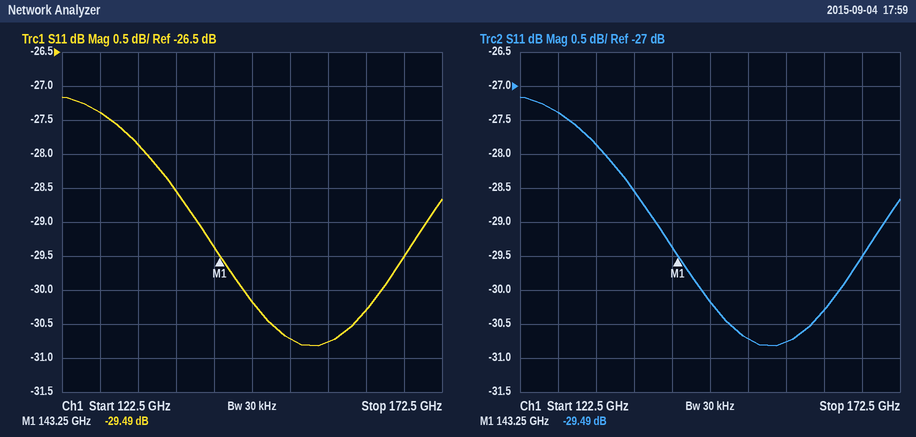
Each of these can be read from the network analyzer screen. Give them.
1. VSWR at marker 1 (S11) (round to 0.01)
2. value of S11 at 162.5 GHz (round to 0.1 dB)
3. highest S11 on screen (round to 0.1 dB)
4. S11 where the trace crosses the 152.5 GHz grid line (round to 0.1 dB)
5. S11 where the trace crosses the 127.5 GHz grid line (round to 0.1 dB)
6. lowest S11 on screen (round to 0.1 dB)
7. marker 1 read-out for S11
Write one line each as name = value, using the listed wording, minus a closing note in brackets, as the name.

VSWR at marker 1 (S11) = 1.07
value of S11 at 162.5 GHz = -30.3 dB
highest S11 on screen = -27.2 dB
S11 where the trace crosses the 152.5 GHz grid line = -30.7 dB
S11 where the trace crosses the 127.5 GHz grid line = -27.4 dB
lowest S11 on screen = -30.8 dB
marker 1 read-out for S11 = -29.49 dB
